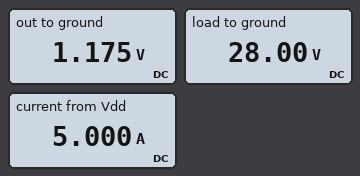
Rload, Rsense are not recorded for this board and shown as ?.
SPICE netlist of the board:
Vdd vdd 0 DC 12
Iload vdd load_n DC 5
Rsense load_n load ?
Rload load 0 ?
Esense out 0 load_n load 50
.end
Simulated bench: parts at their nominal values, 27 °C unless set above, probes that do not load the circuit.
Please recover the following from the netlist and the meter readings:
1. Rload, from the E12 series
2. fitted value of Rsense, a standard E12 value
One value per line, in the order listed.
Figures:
5.6 Ω
4.7 mΩ
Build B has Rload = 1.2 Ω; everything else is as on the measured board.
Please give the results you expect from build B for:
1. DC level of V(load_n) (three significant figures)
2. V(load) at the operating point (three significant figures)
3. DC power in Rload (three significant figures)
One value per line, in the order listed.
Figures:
6.02 V
6.00 V
30.0 W
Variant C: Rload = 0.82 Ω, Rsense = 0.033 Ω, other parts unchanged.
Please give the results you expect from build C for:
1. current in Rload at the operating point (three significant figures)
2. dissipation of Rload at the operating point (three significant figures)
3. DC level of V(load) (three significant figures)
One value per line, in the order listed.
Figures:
5.00 A
20.5 W
4.10 V
